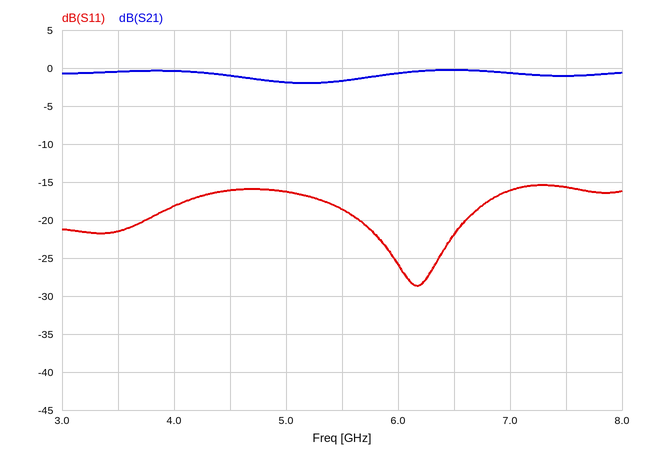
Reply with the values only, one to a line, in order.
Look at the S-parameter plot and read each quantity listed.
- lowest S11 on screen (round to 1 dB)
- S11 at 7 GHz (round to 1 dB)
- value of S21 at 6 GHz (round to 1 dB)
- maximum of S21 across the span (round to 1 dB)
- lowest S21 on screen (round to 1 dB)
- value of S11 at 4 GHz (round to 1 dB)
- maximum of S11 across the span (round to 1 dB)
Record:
-29 dB
-16 dB
-1 dB
0 dB
-2 dB
-18 dB
-15 dB
